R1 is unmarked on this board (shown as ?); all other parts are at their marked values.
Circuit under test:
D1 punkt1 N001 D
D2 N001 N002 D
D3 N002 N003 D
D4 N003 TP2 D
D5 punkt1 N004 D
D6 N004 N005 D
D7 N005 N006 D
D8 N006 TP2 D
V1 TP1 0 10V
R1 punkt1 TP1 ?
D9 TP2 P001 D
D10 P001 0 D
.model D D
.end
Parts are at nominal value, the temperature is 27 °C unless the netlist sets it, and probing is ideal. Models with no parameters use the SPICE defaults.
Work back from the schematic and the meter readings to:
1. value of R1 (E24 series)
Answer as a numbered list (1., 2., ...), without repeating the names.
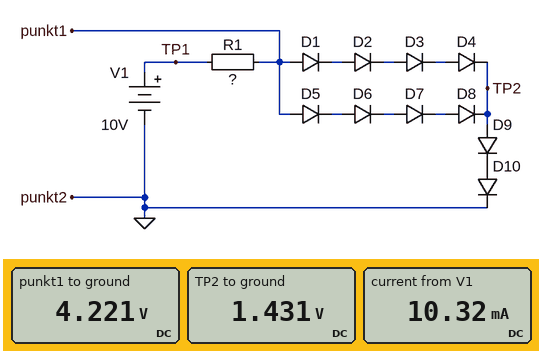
1. 560 Ω
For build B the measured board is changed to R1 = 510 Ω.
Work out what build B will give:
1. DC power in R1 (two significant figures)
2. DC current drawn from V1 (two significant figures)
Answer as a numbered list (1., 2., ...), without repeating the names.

1. 65 mW
2. 11 mA
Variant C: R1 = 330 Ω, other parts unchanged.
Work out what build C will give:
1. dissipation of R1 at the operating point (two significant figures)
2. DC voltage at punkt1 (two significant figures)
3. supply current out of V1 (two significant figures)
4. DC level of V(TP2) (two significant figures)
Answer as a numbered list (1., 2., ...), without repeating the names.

1. 98 mW
2. 4.3 V
3. 17 mA
4. 1.5 V
